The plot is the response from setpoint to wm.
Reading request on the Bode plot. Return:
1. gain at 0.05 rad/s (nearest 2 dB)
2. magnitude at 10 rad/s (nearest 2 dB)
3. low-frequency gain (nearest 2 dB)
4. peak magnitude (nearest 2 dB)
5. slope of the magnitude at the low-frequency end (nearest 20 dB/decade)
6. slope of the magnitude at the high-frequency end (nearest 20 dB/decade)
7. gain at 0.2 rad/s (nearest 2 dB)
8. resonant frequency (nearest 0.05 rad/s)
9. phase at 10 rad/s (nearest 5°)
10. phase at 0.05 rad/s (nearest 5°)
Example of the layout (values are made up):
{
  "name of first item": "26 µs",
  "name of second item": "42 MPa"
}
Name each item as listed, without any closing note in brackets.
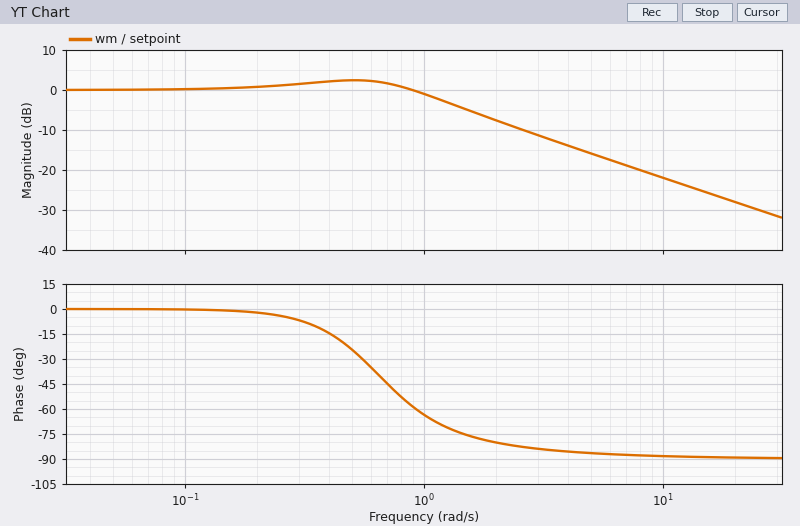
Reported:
{
  "gain at 0.05 rad/s": "0 dB",
  "magnitude at 10 rad/s": "-22 dB",
  "low-frequency gain": "0 dB",
  "peak magnitude": "2 dB",
  "slope of the magnitude at the low-frequency end": "0 dB/decade",
  "slope of the magnitude at the high-frequency end": "-20 dB/decade",
  "gain at 0.2 rad/s": "0 dB",
  "resonant frequency": "0.50 rad/s",
  "phase at 10 rad/s": "-90°",
  "phase at 0.05 rad/s": "0°"
}
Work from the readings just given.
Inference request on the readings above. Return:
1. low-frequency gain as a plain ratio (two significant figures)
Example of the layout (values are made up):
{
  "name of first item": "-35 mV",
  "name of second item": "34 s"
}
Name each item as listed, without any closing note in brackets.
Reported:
{
  "low-frequency gain as a plain ratio": "1.0"
}
